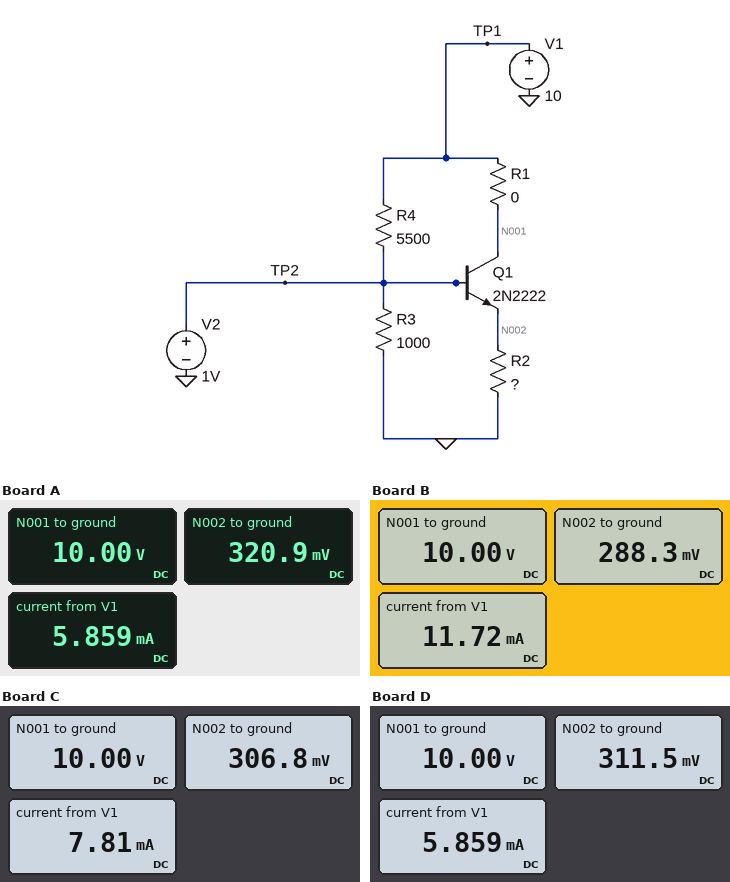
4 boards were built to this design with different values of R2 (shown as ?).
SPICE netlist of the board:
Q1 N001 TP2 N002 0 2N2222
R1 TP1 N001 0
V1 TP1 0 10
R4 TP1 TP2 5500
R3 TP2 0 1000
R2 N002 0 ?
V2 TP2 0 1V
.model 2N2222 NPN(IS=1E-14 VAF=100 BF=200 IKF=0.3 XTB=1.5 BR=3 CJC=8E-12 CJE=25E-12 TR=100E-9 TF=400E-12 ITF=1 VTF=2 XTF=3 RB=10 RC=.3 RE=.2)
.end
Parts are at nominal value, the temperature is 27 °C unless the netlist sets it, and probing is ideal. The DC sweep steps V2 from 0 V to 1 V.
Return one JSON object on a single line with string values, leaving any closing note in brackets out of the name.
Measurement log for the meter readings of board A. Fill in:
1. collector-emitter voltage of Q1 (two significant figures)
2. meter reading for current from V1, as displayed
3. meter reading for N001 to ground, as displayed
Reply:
{"collector-emitter voltage of Q1": "9.7 V", "meter reading for current from V1, as displayed": "5.859 mA", "meter reading for N001 to ground, as displayed": "10.00 V"}
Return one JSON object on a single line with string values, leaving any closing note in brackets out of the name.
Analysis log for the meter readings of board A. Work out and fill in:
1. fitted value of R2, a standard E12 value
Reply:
{"fitted value of R2, a standard E12 value": "120 Ω"}
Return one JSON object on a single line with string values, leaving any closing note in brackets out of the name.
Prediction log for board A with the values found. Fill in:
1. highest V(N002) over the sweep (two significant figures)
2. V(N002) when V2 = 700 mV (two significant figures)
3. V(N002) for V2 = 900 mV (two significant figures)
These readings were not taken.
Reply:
{"highest V(N002) over the sweep": "320 mV", "V(N002) when V2 = 700 mV": "64 mV", "V(N002) for V2 = 900 mV": "230 mV"}
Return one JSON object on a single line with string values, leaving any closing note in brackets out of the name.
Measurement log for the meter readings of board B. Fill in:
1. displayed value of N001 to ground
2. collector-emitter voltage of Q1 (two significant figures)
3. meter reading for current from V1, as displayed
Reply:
{"displayed value of N001 to ground": "10.00 V", "collector-emitter voltage of Q1": "9.7 V", "meter reading for current from V1, as displayed": "11.72 mA"}
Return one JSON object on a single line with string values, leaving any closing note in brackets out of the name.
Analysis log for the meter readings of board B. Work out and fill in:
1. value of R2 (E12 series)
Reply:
{"value of R2": "33 Ω"}
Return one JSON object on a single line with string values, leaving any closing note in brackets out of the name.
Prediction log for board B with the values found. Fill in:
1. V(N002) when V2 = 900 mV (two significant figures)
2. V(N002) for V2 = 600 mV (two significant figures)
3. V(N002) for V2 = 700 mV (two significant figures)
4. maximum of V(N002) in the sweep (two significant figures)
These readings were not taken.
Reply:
{"V(N002) when V2 = 900 mV": "200 mV", "V(N002) for V2 = 600 mV": "3.7 mV", "V(N002) for V2 = 700 mV": "41 mV", "maximum of V(N002) in the sweep": "290 mV"}
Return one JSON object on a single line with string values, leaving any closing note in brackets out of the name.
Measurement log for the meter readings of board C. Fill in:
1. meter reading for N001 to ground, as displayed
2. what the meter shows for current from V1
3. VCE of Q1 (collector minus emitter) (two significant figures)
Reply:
{"meter reading for N001 to ground, as displayed": "10.00 V", "what the meter shows for current from V1": "7.81 mA", "VCE of Q1 (collector minus emitter)": "9.7 V"}
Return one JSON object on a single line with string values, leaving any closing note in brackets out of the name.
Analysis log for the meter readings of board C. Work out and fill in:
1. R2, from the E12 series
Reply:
{"R2, from the E12 series": "68 Ω"}
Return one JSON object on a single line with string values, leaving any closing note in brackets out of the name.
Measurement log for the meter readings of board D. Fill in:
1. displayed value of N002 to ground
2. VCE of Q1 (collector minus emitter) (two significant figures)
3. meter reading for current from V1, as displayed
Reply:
{"displayed value of N002 to ground": "311.5 mV", "VCE of Q1 (collector minus emitter)": "9.7 V", "meter reading for current from V1, as displayed": "5.859 mA"}
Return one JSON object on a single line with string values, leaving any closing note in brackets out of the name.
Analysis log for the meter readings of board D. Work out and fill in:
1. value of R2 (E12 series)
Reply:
{"value of R2": "82 Ω"}
